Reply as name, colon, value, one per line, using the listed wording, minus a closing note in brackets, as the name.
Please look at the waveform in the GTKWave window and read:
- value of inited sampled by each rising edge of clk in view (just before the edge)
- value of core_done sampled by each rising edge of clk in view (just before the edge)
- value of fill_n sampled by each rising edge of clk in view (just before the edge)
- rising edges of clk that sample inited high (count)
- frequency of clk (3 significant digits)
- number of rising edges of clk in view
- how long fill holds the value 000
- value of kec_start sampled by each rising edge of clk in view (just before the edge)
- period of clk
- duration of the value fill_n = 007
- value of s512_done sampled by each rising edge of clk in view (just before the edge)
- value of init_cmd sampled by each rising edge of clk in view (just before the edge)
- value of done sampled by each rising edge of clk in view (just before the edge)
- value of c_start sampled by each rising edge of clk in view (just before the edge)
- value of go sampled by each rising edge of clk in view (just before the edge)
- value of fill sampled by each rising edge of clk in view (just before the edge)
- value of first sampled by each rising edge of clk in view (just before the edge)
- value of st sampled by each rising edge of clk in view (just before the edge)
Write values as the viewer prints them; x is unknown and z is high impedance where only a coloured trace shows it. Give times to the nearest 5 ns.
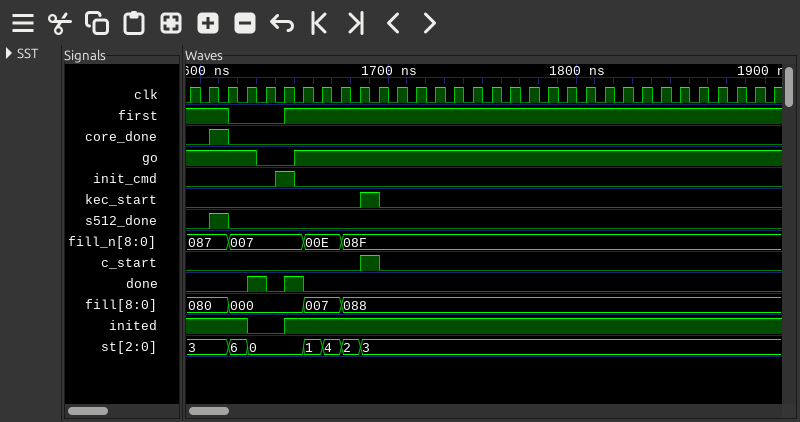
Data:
value of inited sampled by each rising edge of clk in view: 1 1 1 1 0 0 1 1 1 1 1 1 1 1 1 1 1 1 1 1 1 1 1 1 1 1 1 1 1 1 1 1
value of core_done sampled by each rising edge of clk in view: 0 0 1 0 0 0 0 0 0 0 0 0 0 0 0 0 0 0 0 0 0 0 0 0 0 0 0 0 0 0 0 0
value of fill_n sampled by each rising edge of clk in view: 087, 087, 087, 007, 007, 007, 007, 00E, 00E, 08F, 08F, 08F, 08F, 08F, 08F, 08F, 08F, 08F, 08F, 08F, 08F, 08F, 08F, 08F, 08F, 08F, 08F, 08F, 08F, 08F, 08F, 08F
rising edges of clk that sample inited high: 30
frequency of clk: 100 MHz
number of rising edges of clk in view: 32
how long fill holds the value 000: 40 ns
value of kec_start sampled by each rising edge of clk in view: 0 0 0 0 0 0 0 0 0 0 1 0 0 0 0 0 0 0 0 0 0 0 0 0 0 0 0 0 0 0 0 0
period of clk: 10 ns
duration of the value fill_n = 007: 40 ns
value of s512_done sampled by each rising edge of clk in view: 0 0 1 0 0 0 0 0 0 0 0 0 0 0 0 0 0 0 0 0 0 0 0 0 0 0 0 0 0 0 0 0
value of init_cmd sampled by each rising edge of clk in view: 0 0 0 0 0 1 0 0 0 0 0 0 0 0 0 0 0 0 0 0 0 0 0 0 0 0 0 0 0 0 0 0
value of done sampled by each rising edge of clk in view: 0 0 0 0 1 0 1 0 0 0 0 0 0 0 0 0 0 0 0 0 0 0 0 0 0 0 0 0 0 0 0 0
value of c_start sampled by each rising edge of clk in view: 0 0 0 0 0 0 0 0 0 0 1 0 0 0 0 0 0 0 0 0 0 0 0 0 0 0 0 0 0 0 0 0
value of go sampled by each rising edge of clk in view: 1 1 1 1 0 0 1 1 1 1 1 1 1 1 1 1 1 1 1 1 1 1 1 1 1 1 1 1 1 1 1 1
value of fill sampled by each rising edge of clk in view: 080, 080, 080, 000, 000, 000, 000, 007, 007, 088, 088, 088, 088, 088, 088, 088, 088, 088, 088, 088, 088, 088, 088, 088, 088, 088, 088, 088, 088, 088, 088, 088
value of first sampled by each rising edge of clk in view: 1 1 1 0 0 0 1 1 1 1 1 1 1 1 1 1 1 1 1 1 1 1 1 1 1 1 1 1 1 1 1 1
value of st sampled by each rising edge of clk in view: 3, 3, 3, 6, 0, 0, 0, 1, 4, 2, 3, 3, 3, 3, 3, 3, 3, 3, 3, 3, 3, 3, 3, 3, 3, 3, 3, 3, 3, 3, 3, 3
